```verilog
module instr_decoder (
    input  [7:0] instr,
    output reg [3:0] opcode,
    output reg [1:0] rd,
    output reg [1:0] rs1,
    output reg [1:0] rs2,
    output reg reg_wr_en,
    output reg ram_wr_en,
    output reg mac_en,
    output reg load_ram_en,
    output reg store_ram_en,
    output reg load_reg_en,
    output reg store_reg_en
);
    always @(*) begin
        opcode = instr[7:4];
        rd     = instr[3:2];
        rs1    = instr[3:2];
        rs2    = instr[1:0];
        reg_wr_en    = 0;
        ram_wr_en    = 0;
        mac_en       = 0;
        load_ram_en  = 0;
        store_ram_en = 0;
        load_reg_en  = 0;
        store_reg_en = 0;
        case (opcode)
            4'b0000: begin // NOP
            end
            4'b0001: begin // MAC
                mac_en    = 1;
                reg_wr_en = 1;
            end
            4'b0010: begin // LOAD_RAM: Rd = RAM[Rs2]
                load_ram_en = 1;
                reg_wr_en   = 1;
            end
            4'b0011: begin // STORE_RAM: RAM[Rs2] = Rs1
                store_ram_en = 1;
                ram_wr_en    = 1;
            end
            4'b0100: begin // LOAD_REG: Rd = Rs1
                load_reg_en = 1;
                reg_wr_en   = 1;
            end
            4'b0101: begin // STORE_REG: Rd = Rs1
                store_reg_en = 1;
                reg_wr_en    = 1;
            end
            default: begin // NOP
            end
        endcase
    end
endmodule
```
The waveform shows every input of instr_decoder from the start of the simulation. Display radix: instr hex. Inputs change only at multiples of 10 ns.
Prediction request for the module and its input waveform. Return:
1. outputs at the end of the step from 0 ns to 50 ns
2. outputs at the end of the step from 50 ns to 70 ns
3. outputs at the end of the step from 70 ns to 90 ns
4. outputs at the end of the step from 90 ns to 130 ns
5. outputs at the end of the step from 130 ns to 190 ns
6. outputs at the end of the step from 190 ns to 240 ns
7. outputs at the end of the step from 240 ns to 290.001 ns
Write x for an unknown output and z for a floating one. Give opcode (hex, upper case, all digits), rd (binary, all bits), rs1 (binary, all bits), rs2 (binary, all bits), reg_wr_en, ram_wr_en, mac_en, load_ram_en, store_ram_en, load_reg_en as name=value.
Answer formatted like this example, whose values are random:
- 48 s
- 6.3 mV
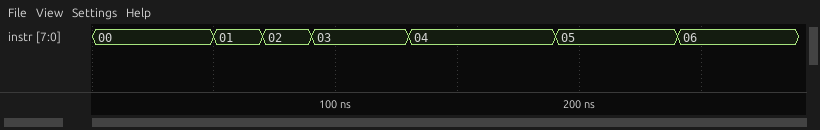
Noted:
- opcode=0, rd=00, rs1=00, rs2=00, reg_wr_en=0, ram_wr_en=0, mac_en=0, load_ram_en=0, store_ram_en=0, load_reg_en=0
- opcode=0, rd=00, rs1=00, rs2=01, reg_wr_en=0, ram_wr_en=0, mac_en=0, load_ram_en=0, store_ram_en=0, load_reg_en=0
- opcode=0, rd=00, rs1=00, rs2=10, reg_wr_en=0, ram_wr_en=0, mac_en=0, load_ram_en=0, store_ram_en=0, load_reg_en=0
- opcode=0, rd=00, rs1=00, rs2=11, reg_wr_en=0, ram_wr_en=0, mac_en=0, load_ram_en=0, store_ram_en=0, load_reg_en=0
- opcode=0, rd=01, rs1=01, rs2=00, reg_wr_en=0, ram_wr_en=0, mac_en=0, load_ram_en=0, store_ram_en=0, load_reg_en=0
- opcode=0, rd=01, rs1=01, rs2=01, reg_wr_en=0, ram_wr_en=0, mac_en=0, load_ram_en=0, store_ram_en=0, load_reg_en=0
- opcode=0, rd=01, rs1=01, rs2=10, reg_wr_en=0, ram_wr_en=0, mac_en=0, load_ram_en=0, store_ram_en=0, load_reg_en=0
